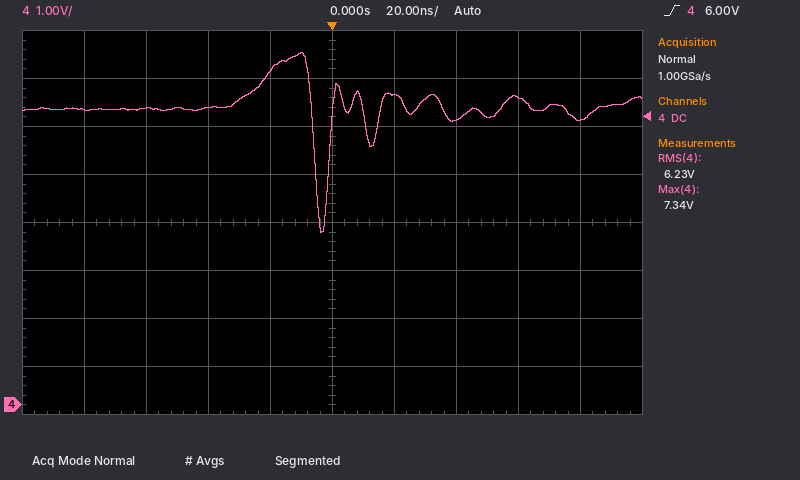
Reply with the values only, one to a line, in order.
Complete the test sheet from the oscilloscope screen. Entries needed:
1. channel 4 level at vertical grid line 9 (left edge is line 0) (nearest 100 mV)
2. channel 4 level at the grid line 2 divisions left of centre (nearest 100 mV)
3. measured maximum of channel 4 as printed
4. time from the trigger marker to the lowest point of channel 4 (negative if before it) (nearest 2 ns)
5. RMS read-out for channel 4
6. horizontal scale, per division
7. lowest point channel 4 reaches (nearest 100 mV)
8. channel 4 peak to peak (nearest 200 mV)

5.9 V
6.2 V
7.34 V
-4 ns
6.23 V
20 ns
3.6 V
3.8 V
